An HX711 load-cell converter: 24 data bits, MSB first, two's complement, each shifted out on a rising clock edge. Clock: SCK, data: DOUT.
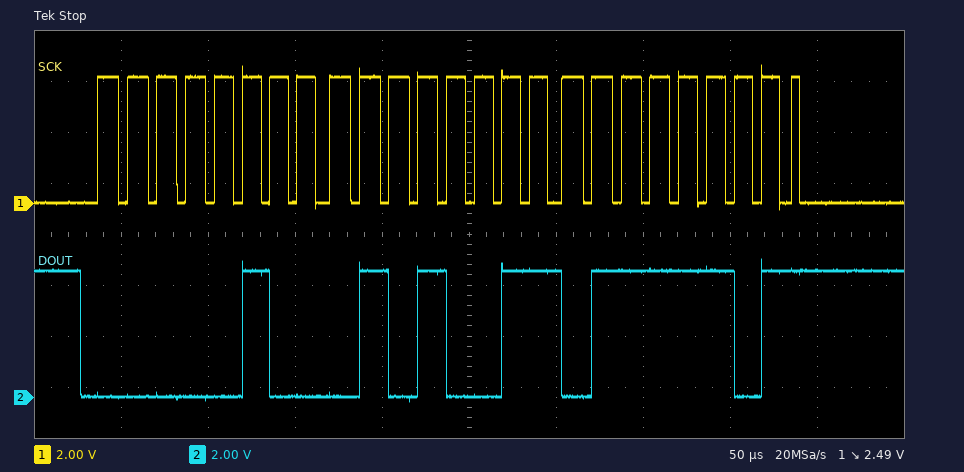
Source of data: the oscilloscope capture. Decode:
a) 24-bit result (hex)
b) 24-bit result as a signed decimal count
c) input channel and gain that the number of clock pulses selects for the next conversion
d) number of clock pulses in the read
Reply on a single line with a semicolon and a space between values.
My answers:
0x04537D; 283517; channel A, gain 128; 25
